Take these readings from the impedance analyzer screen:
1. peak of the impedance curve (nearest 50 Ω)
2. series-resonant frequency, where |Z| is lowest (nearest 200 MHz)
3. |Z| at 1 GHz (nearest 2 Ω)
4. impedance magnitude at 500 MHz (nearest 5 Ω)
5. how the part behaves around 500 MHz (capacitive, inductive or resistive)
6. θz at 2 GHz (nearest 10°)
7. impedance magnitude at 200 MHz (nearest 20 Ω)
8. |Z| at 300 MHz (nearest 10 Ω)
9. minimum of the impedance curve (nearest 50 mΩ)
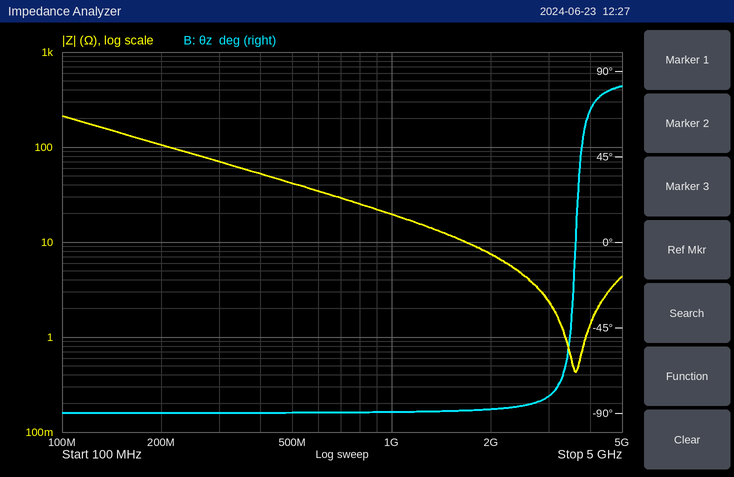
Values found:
200 Ω
3.6 GHz
20 Ω
40 Ω
capacitive
-90°
100 Ω
70 Ω
450 mΩ
